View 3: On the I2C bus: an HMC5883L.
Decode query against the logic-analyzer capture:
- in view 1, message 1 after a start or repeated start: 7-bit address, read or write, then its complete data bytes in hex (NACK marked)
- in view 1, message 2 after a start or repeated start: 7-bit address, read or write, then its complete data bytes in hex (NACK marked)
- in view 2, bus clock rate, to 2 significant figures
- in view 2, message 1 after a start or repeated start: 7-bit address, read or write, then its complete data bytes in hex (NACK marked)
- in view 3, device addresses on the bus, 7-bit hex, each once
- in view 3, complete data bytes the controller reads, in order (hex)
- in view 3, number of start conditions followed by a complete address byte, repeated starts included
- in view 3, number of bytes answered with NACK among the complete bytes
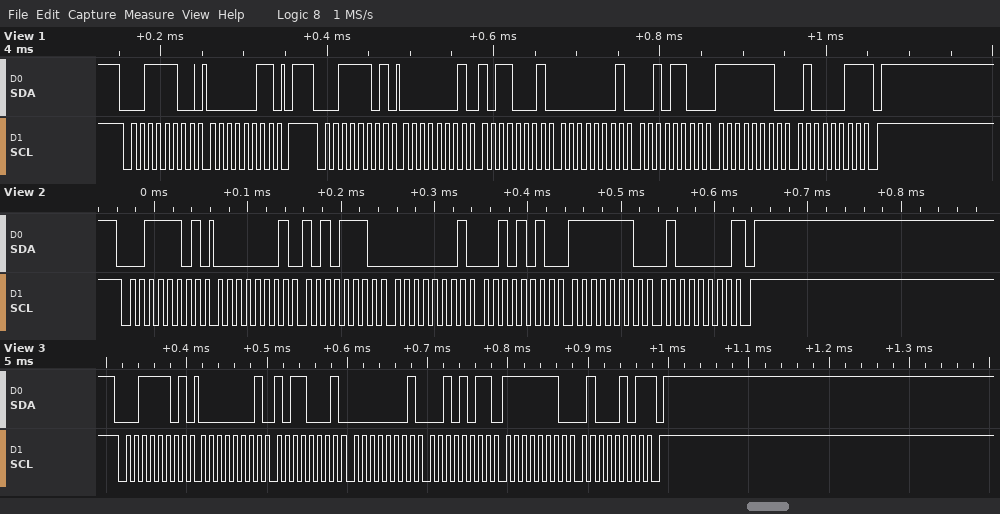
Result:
0x1E write: 03
0x1E read: 01 B1 01 2C FE 43 NACK
100 kHz
0x1E read: 01 AE 01 2A FE 40 NACK
0x1E
01 B1 01 2B FE 45
1
1
